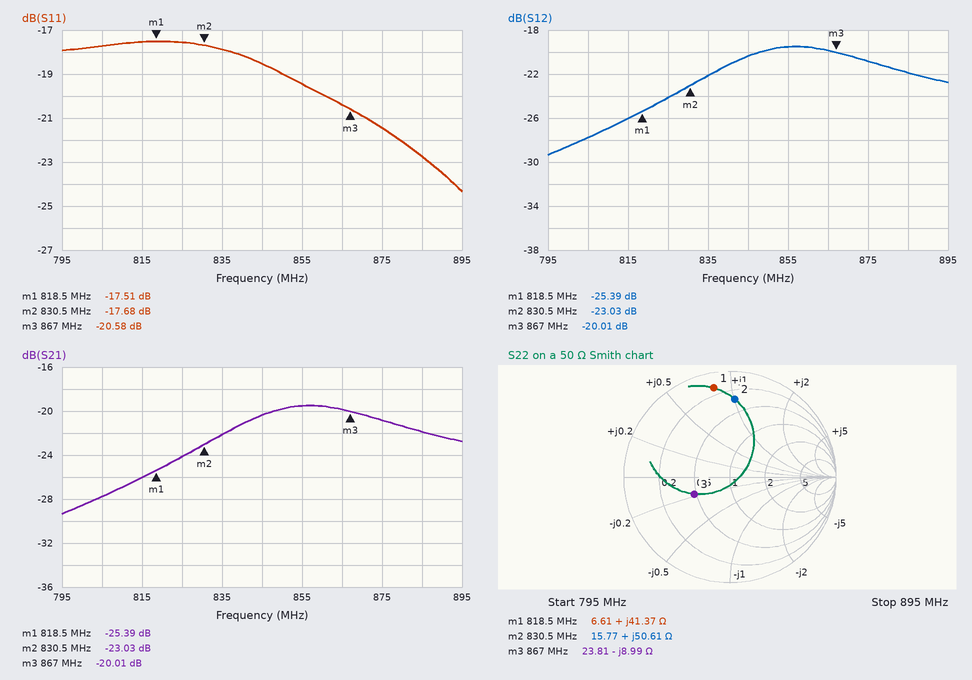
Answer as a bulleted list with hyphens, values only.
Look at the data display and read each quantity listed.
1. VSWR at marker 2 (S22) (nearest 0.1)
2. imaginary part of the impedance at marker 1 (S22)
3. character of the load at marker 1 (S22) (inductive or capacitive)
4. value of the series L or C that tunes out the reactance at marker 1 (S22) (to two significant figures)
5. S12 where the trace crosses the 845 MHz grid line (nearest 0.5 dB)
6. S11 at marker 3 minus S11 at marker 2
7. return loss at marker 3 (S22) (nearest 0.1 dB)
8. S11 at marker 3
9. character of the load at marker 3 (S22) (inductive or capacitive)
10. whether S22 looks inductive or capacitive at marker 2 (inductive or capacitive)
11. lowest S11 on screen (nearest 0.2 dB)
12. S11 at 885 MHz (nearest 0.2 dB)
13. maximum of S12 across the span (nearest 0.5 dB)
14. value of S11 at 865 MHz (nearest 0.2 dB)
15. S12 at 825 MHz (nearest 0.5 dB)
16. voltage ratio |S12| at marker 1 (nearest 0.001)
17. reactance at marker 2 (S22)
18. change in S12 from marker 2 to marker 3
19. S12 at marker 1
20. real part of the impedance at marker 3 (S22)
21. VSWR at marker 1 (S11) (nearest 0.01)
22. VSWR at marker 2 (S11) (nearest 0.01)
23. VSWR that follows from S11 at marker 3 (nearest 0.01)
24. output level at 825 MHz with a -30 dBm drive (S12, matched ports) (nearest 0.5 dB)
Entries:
- 6.6
- +41.37 Ω
- inductive
- 4.7 pF
- -20.5 dB
- -2.90 dB
- 8.6 dB
- -20.58 dB
- capacitive
- inductive
- -24.4 dB
- -22.8 dB
- -19.5 dB
- -20.4 dB
- -24.0 dB
- 0.054
- +50.61 Ω
- 3.02 dB
- -25.39 dB
- 23.81 Ω
- 1.31
- 1.30
- 1.21
- -54.0 dBm
